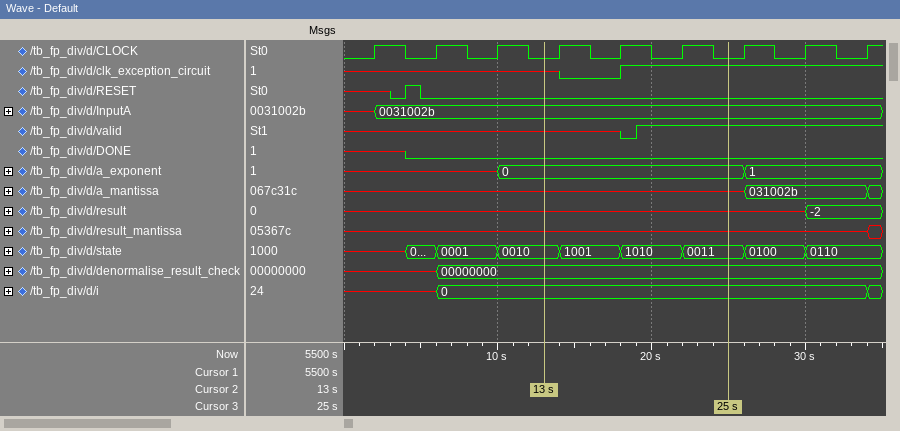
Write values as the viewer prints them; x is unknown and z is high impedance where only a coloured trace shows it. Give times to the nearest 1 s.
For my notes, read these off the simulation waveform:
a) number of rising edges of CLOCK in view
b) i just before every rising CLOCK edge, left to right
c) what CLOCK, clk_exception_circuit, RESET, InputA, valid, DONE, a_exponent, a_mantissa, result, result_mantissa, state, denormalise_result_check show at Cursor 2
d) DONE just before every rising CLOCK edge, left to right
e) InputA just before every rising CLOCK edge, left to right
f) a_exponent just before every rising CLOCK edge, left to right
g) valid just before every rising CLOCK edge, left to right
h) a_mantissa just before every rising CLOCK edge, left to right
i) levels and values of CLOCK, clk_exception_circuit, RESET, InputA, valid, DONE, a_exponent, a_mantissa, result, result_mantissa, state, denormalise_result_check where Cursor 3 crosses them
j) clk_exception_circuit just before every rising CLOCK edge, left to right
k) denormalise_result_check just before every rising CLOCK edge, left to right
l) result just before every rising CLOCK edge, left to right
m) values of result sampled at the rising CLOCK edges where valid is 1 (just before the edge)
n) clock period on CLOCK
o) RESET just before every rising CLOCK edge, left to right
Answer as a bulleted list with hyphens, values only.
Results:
- 9
- x, x, 0, 0, 0, 0, 0, 0, 0
- CLOCK=0, clk_exception_circuit=x, RESET=0, InputA=0031002b, valid=x, DONE=0, a_exponent=0, a_mantissa=x, result=x, result_mantissa=x, state=0010, denormalise_result_check=00000000
- x 0 0 0 0 0 0 0 0
- x, 0031002b, 0031002b, 0031002b, 0031002b, 0031002b, 0031002b, 0031002b, 0031002b
- x, x, x, 0, 0, 0, 0, 1, 1
- x x x x x 1 1 1 1
- x, x, x, x, x, x, x, 031002b, 031002b
- CLOCK=0, clk_exception_circuit=1, RESET=0, InputA=0031002b, valid=1, DONE=0, a_exponent=0, a_mantissa=x, result=x, result_mantissa=x, state=0011, denormalise_result_check=00000000
- x x x x 0 1 1 1 1
- x, x, 00000000, 00000000, 00000000, 00000000, 00000000, 00000000, 00000000
- x, x, x, x, x, x, x, x, -2
- x, x, x, -2
- 4 s
- x 0 0 0 0 0 0 0 0
